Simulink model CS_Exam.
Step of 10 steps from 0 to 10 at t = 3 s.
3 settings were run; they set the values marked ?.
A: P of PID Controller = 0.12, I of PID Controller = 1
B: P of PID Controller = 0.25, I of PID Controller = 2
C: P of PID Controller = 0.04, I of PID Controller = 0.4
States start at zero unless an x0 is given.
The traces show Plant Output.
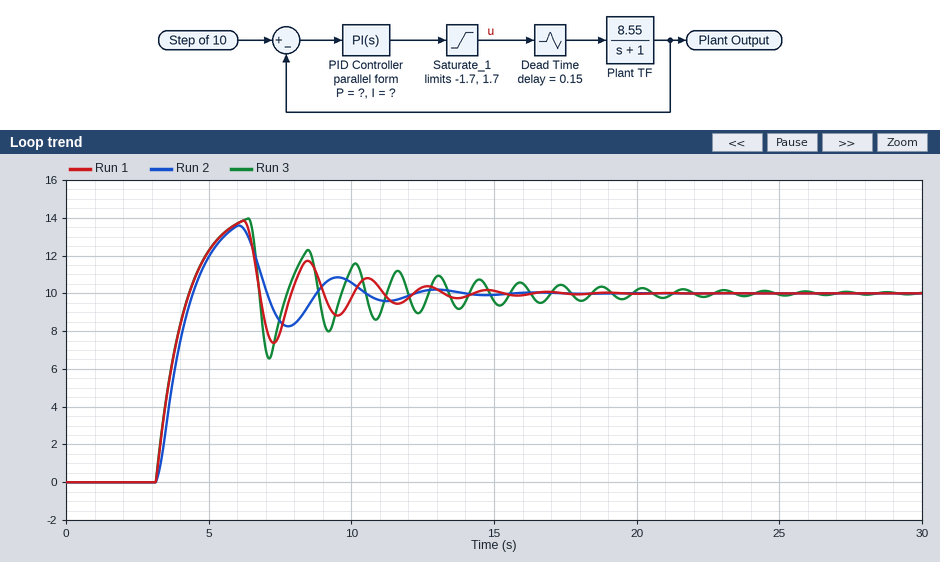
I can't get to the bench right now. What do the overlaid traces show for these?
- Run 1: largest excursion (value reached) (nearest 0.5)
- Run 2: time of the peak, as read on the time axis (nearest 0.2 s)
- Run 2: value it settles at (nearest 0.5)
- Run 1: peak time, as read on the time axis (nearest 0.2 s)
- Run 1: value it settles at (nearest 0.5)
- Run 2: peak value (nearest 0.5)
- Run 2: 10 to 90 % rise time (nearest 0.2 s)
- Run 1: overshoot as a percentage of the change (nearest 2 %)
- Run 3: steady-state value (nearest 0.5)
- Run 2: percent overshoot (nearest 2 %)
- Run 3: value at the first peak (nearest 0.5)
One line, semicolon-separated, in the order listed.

14.0; 6.0 s; 10.0; 6.2 s; 10.0; 13.5; 1.0 s; 38 %; 10.0; 36 %; 14.0
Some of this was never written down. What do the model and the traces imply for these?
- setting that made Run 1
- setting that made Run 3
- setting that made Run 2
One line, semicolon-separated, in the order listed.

A; B; C
